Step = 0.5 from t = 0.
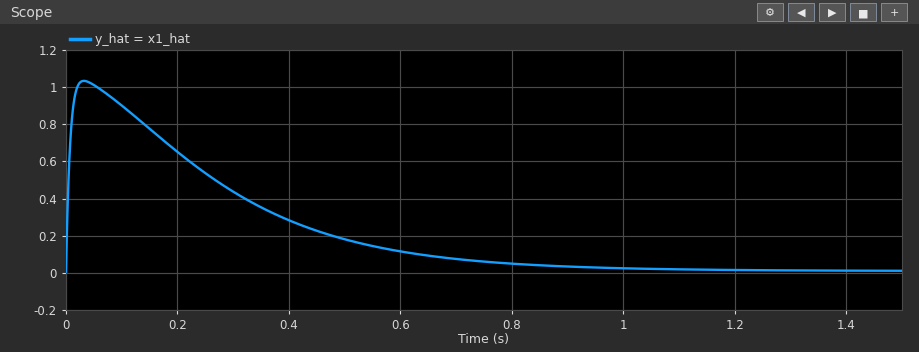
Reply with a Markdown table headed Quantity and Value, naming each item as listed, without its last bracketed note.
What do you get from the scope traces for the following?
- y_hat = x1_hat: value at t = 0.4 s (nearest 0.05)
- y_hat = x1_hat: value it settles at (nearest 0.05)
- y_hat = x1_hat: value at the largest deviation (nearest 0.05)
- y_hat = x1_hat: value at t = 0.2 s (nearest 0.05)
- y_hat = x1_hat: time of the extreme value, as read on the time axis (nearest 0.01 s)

| Quantity | Value |
|---|---|
| y_hat = x1_hat: value at t = 0.4 s | 0.30 |
| y_hat = x1_hat: value it settles at | 0.00 |
| y_hat = x1_hat: value at the largest deviation | 1.05 |
| y_hat = x1_hat: value at t = 0.2 s | 0.65 |
| y_hat = x1_hat: time of the extreme value, as read on the time axis | 0.03 s |
